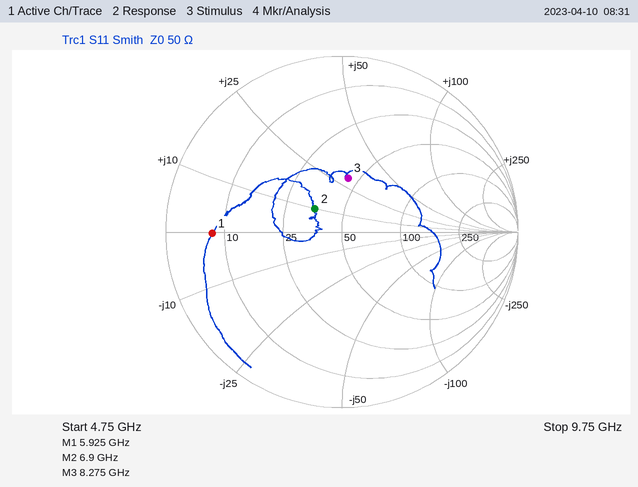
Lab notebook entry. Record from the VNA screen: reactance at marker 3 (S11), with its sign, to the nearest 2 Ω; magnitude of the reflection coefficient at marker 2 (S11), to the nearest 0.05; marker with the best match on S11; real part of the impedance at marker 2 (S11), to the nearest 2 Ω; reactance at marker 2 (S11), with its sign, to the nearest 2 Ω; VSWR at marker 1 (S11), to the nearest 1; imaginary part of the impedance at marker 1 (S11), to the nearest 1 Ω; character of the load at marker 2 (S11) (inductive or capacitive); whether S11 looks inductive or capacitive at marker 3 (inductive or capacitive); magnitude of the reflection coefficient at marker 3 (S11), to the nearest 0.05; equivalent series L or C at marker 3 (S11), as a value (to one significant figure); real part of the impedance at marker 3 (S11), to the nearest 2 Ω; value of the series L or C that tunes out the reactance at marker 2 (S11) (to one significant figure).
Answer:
+30 Ω
0.20
marker 2
36 Ω
+10 Ω
7
0 Ω
inductive
inductive
0.30
600 pH
44 Ω
2 pF
